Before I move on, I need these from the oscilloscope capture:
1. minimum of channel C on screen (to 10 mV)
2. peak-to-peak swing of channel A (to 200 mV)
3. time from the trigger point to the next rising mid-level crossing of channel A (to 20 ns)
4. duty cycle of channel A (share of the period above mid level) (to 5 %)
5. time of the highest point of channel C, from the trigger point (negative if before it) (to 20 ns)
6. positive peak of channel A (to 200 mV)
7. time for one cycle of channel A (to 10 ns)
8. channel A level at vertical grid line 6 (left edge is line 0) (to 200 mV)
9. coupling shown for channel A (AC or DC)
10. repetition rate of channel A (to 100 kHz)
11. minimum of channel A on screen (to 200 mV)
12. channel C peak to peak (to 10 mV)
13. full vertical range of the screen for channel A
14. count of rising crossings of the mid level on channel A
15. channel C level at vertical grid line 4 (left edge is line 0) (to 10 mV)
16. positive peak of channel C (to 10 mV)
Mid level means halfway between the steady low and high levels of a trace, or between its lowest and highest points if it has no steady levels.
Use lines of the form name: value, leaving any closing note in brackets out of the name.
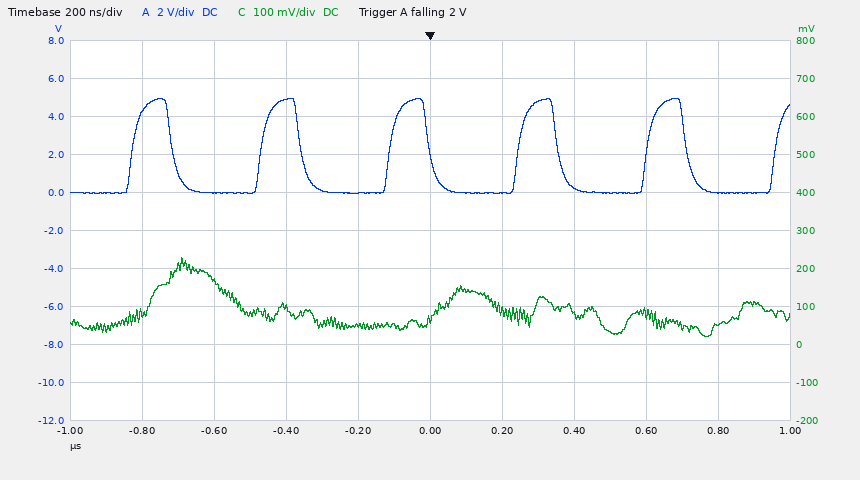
minimum of channel C on screen: 20 mV
peak-to-peak swing of channel A: 5.0 V
time from the trigger point to the next rising mid-level crossing of channel A: 240 ns
duty cycle of channel A (share of the period above mid level): 30 %
time of the highest point of channel C, from the trigger point (negative if before it): -680 ns
positive peak of channel A: 5.0 V
time for one cycle of channel A: 360 ns
channel A level at vertical grid line 6 (left edge is line 0): 0.0 V
coupling shown for channel A: DC
repetition rate of channel A: 2.8 MHz
minimum of channel A on screen: 0.0 V
channel C peak to peak: 210 mV
full vertical range of the screen for channel A: 20 V
count of rising crossings of the mid level on channel A: 6
channel C level at vertical grid line 4 (left edge is line 0): 50 mV
positive peak of channel C: 230 mV
